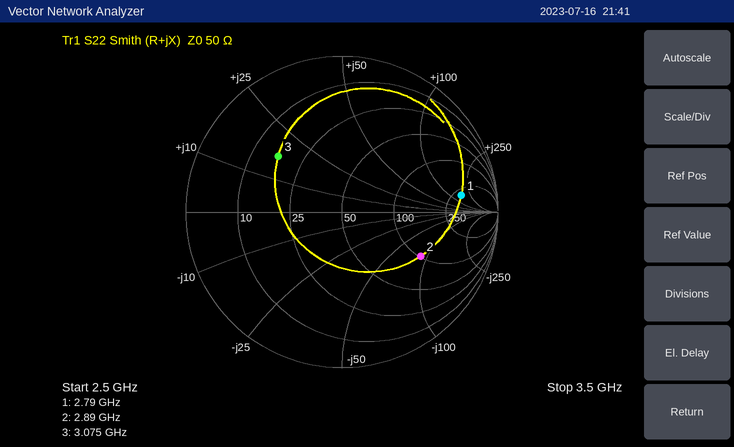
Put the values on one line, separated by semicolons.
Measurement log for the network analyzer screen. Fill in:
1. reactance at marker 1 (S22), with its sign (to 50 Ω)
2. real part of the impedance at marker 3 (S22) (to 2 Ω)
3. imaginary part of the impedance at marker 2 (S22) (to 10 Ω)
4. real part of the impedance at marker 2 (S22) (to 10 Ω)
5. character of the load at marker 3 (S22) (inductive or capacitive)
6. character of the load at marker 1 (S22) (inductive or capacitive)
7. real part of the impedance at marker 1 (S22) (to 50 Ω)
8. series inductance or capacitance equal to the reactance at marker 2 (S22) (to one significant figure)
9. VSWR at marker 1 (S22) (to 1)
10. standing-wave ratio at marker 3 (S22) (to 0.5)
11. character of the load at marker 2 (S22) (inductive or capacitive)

+150 Ω; 16 Ω; -90 Ω; 100 Ω; inductive; inductive; 300 Ω; 600 fF; 8; 3.5; capacitive
